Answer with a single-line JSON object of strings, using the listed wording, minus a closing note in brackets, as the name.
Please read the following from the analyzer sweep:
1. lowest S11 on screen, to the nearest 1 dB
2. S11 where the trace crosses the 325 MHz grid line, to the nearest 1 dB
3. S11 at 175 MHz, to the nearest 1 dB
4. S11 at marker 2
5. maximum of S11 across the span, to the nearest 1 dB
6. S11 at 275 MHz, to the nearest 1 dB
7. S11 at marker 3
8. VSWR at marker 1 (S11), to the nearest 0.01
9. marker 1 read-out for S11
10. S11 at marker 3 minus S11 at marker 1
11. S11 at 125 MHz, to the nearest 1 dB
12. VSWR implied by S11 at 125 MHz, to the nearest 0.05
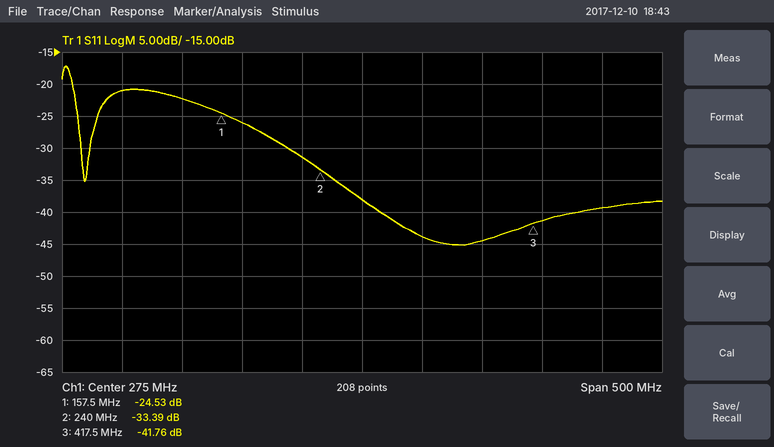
{"lowest S11 on screen, to the nearest 1 dB": "-45 dB", "S11 where the trace crosses the 325 MHz grid line, to the nearest 1 dB": "-44 dB", "S11 at 175 MHz, to the nearest 1 dB": "-26 dB", "S11 at marker 2": "-33.39 dB", "maximum of S11 across the span, to the nearest 1 dB": "-17 dB", "S11 at 275 MHz, to the nearest 1 dB": "-38 dB", "S11 at marker 3": "-41.76 dB", "VSWR at marker 1 (S11), to the nearest 0.01": "1.13", "marker 1 read-out for S11": "-24.53 dB", "S11 at marker 3 minus S11 at marker 1": "-17.23 dB", "S11 at 125 MHz, to the nearest 1 dB": "-22 dB", "VSWR implied by S11 at 125 MHz, to the nearest 0.05": "1.15"}
